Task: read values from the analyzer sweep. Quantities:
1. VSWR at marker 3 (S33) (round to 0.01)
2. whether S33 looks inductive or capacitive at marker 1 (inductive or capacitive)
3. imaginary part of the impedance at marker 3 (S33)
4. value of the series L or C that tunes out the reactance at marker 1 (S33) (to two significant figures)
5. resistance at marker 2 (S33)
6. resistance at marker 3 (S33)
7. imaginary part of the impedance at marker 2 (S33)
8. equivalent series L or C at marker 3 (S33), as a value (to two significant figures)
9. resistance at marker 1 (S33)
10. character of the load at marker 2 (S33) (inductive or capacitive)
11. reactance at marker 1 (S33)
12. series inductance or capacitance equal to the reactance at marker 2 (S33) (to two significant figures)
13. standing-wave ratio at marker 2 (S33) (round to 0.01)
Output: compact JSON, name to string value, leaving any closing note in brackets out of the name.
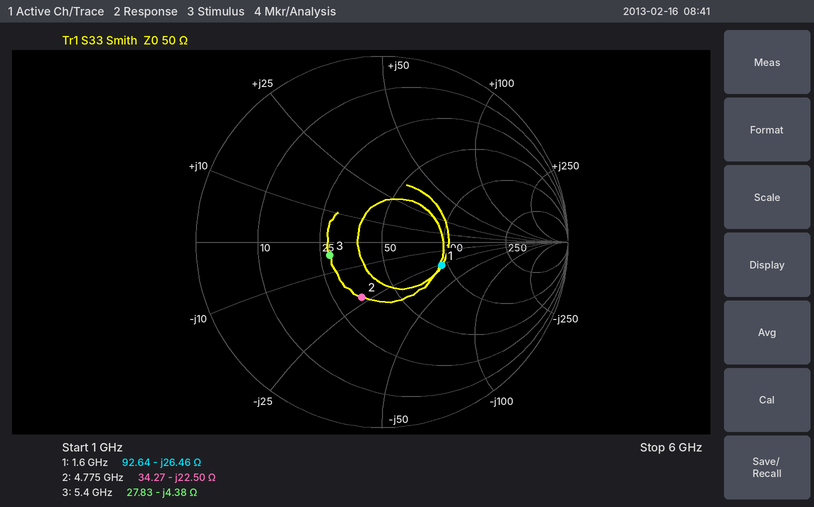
{"VSWR at marker 3 (S33)": "1.82", "whether S33 looks inductive or capacitive at marker 1": "capacitive", "imaginary part of the impedance at marker 3": "-4.38 Ω", "value of the series L or C that tunes out the reactance at marker 1 (S33)": "2.6 nH", "resistance at marker 2": "34.27 Ω", "resistance at marker 3": "27.83 Ω", "imaginary part of the impedance at marker 2": "-22.50 Ω", "equivalent series L or C at marker 3 (S33), as a value": "6.7 pF", "resistance at marker 1": "92.64 Ω", "character of the load at marker 2 (S33)": "capacitive", "reactance at marker 1": "-26.46 Ω", "series inductance or capacitance equal to the reactance at marker 2 (S33)": "1.5 pF", "standing-wave ratio at marker 2 (S33)": "1.92"}
